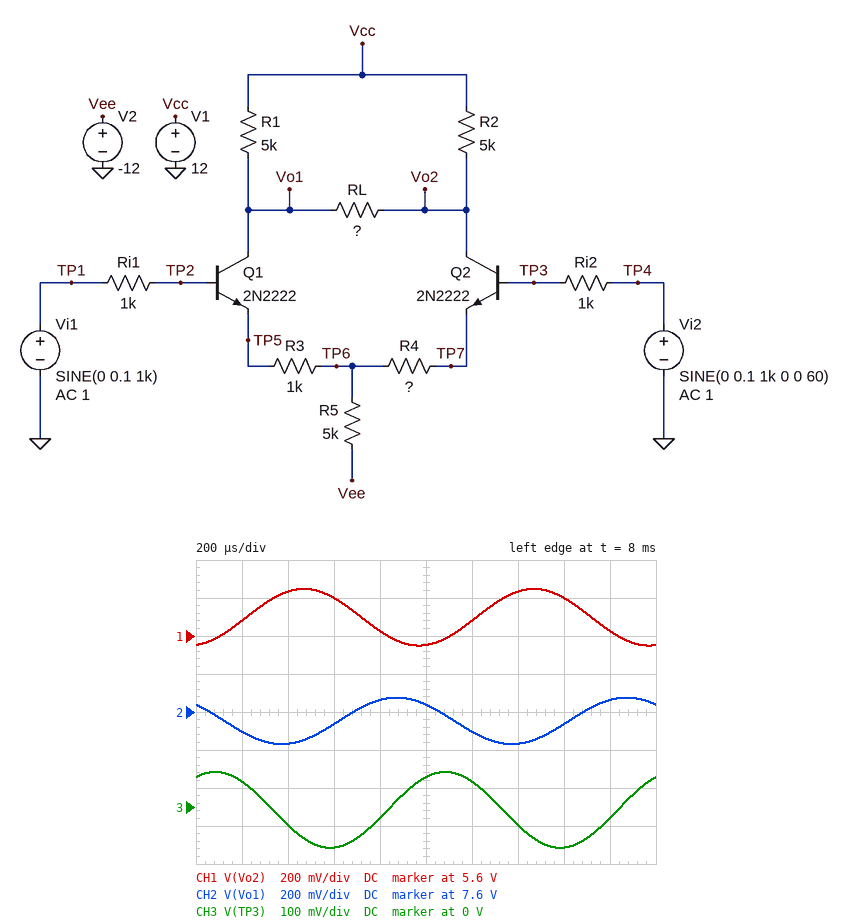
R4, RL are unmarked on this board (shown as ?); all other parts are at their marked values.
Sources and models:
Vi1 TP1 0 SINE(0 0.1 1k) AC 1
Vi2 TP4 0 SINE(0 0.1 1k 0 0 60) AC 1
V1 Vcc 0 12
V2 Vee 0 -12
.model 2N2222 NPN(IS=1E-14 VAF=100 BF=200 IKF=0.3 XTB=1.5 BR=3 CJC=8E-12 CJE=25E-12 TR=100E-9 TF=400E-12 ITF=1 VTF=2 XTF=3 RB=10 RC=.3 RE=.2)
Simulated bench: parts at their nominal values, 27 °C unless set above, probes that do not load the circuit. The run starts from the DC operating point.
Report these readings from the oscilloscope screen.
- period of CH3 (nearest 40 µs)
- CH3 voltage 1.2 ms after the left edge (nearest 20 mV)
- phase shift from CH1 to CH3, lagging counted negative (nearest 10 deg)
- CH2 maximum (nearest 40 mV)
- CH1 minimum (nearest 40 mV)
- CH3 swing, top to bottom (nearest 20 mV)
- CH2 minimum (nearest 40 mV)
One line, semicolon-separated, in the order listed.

1.00 ms; 60 mV; 140 deg; 7.68 V; 5.56 V; 200 mV; 7.44 V
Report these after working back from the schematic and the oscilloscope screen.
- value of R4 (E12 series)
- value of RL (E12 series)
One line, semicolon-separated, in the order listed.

330 Ω; 5.6 kΩ
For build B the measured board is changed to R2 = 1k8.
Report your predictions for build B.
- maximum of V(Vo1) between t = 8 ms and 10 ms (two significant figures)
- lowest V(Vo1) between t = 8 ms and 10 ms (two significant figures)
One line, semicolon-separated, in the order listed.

9.3 V; 9.0 V
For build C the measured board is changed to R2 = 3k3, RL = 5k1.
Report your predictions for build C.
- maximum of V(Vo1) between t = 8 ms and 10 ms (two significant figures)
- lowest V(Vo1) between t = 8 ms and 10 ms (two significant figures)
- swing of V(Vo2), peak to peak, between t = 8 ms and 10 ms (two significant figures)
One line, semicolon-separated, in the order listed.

8.4 V; 8.2 V; 210 mV
